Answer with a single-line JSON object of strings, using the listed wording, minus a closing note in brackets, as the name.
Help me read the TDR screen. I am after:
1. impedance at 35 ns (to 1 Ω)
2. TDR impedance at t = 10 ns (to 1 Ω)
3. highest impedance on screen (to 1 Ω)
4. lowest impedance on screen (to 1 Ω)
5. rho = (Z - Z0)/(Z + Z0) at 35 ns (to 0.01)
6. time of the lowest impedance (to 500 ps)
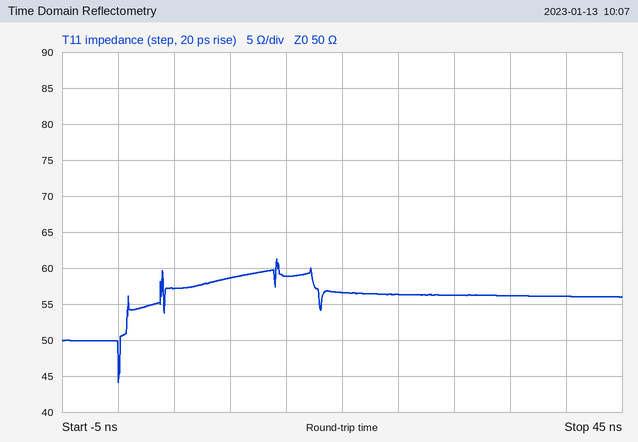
{"impedance at 35 ns": "56 Ω", "TDR impedance at t = 10 ns": "59 Ω", "highest impedance on screen": "61 Ω", "lowest impedance on screen": "44 Ω", "rho = (Z - Z0)/(Z + Z0) at 35 ns": "+0.06", "time of the lowest impedance": "0.0 ns"}
